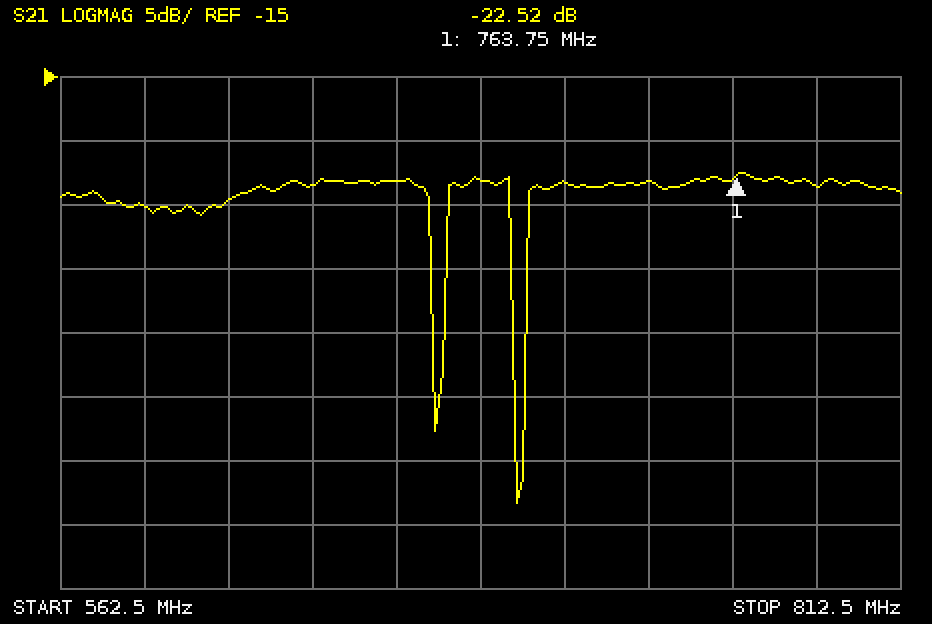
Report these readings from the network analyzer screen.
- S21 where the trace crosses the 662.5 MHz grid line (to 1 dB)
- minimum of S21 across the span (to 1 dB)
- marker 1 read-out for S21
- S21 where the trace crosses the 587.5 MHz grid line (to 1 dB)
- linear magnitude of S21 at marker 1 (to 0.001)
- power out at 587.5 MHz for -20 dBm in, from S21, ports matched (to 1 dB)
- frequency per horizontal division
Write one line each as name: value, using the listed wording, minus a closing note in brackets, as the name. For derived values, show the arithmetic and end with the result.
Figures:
S21 where the trace crosses the 662.5 MHz grid line: -23 dB
minimum of S21 across the span: -48 dB
marker 1 read-out for S21: -22.52 dB
S21 where the trace crosses the 587.5 MHz grid line: -25 dB
linear magnitude of S21 at marker 1: 10^(-22.52/20) ≈ 0.075
power out at 587.5 MHz for -20 dBm in, from S21, ports matched: -20 dBm + (-25 dB) = -45 dBm
frequency per horizontal division: 25 MHz
